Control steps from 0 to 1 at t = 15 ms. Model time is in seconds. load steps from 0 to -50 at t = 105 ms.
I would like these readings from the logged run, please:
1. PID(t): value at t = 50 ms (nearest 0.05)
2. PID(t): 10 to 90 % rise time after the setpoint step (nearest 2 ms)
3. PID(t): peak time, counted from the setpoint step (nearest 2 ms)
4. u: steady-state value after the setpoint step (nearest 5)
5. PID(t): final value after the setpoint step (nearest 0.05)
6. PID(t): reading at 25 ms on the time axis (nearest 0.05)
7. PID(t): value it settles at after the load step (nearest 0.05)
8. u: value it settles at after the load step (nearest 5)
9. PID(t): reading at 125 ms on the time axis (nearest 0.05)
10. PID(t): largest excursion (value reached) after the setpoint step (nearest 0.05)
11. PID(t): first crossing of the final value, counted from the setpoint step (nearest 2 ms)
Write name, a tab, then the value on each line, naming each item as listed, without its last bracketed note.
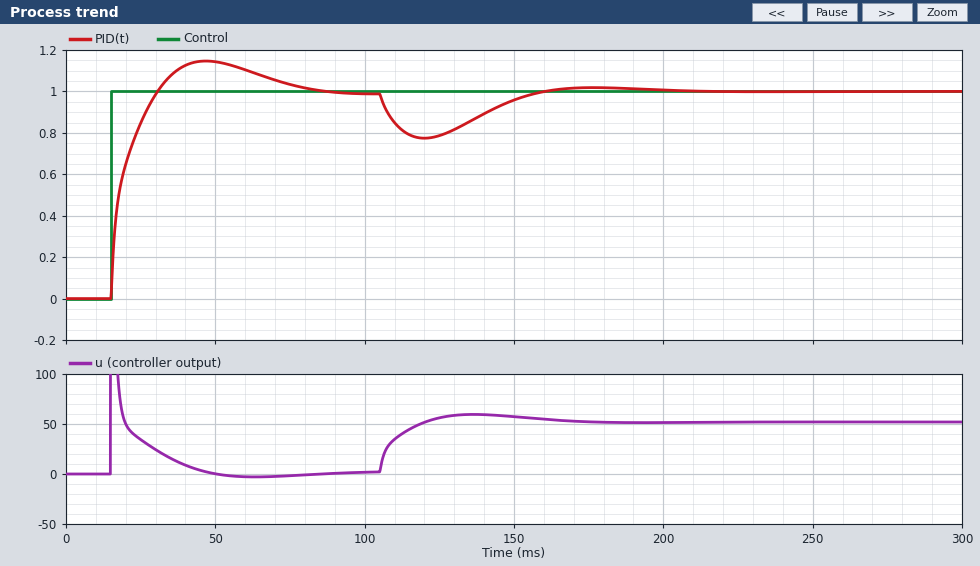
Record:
PID(t): value at t = 50 ms	1.15
PID(t): 10 to 90 % rise time after the setpoint step	12 ms
PID(t): peak time, counted from the setpoint step	32 ms
u: steady-state value after the setpoint step	0
PID(t): final value after the setpoint step	1.00
PID(t): reading at 25 ms on the time axis	0.85
PID(t): value it settles at after the load step	1.00
u: value it settles at after the load step	50
PID(t): reading at 125 ms on the time axis	0.80
PID(t): largest excursion (value reached) after the setpoint step	1.15
PID(t): first crossing of the final value, counted from the setpoint step	16 ms
